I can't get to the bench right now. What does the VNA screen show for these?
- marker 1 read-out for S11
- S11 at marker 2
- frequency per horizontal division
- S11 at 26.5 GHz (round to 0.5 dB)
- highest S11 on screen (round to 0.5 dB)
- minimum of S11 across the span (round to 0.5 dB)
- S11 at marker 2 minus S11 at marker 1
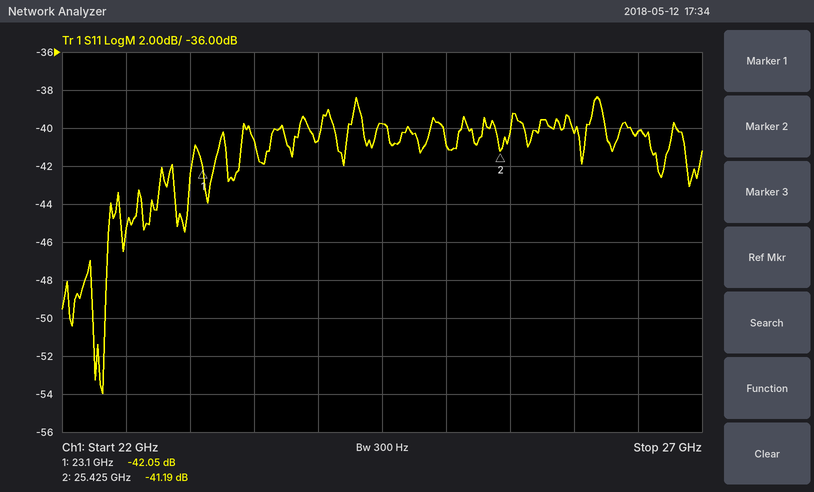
-42.05 dB
-41.19 dB
500 MHz
-40.0 dB
-38.5 dB
-54.0 dB
0.86 dB
